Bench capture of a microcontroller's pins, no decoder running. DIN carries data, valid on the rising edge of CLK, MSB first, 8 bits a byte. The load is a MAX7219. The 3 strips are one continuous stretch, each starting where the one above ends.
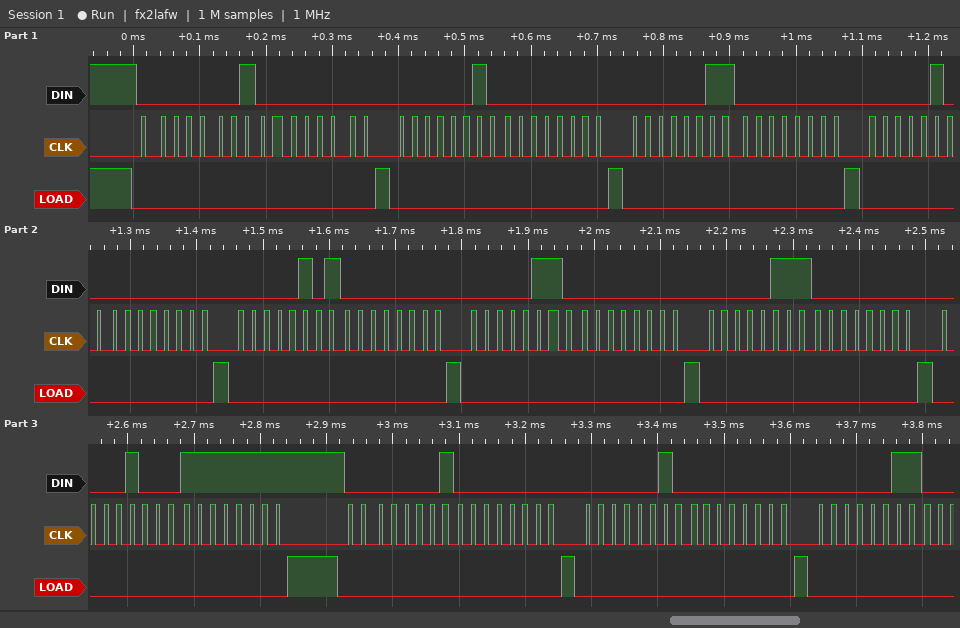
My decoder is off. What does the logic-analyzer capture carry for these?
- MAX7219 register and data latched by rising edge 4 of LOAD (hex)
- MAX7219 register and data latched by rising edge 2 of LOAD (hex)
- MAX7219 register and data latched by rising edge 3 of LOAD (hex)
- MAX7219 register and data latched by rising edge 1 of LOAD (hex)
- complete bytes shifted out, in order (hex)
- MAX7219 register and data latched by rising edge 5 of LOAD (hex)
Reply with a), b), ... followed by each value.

a) register 0x4, data 0x00
b) register 0x2, data 0x00
c) register 0x3, data 0x00
d) register 0x1, data 0x00
e) 01 00 02 00 03 00 04 00 05 00 06 00 07 00 08 FF 01 00 02 00 03
f) register 0x5, data 0x00
